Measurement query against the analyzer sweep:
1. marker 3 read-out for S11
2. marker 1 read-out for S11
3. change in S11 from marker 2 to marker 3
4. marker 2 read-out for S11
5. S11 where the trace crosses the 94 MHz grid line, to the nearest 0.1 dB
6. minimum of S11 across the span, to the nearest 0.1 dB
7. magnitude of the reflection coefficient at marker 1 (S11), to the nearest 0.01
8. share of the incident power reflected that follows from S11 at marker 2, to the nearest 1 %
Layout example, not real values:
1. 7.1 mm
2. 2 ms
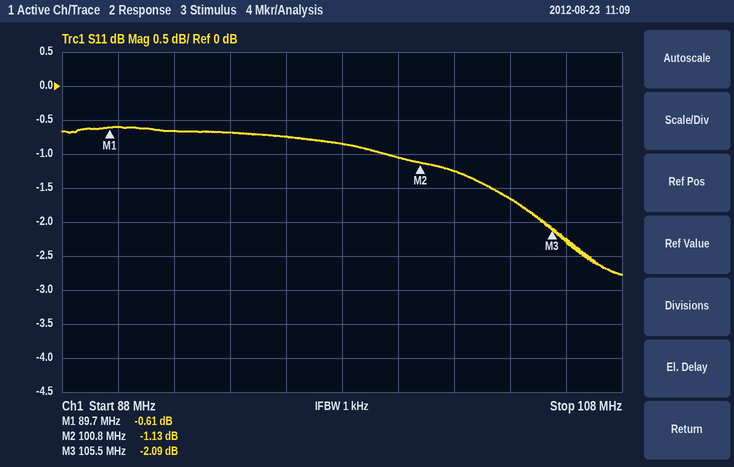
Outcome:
1. -2.09 dB
2. -0.61 dB
3. -0.96 dB
4. -1.13 dB
5. -0.7 dB
6. -2.8 dB
7. 0.93
8. 77 %
